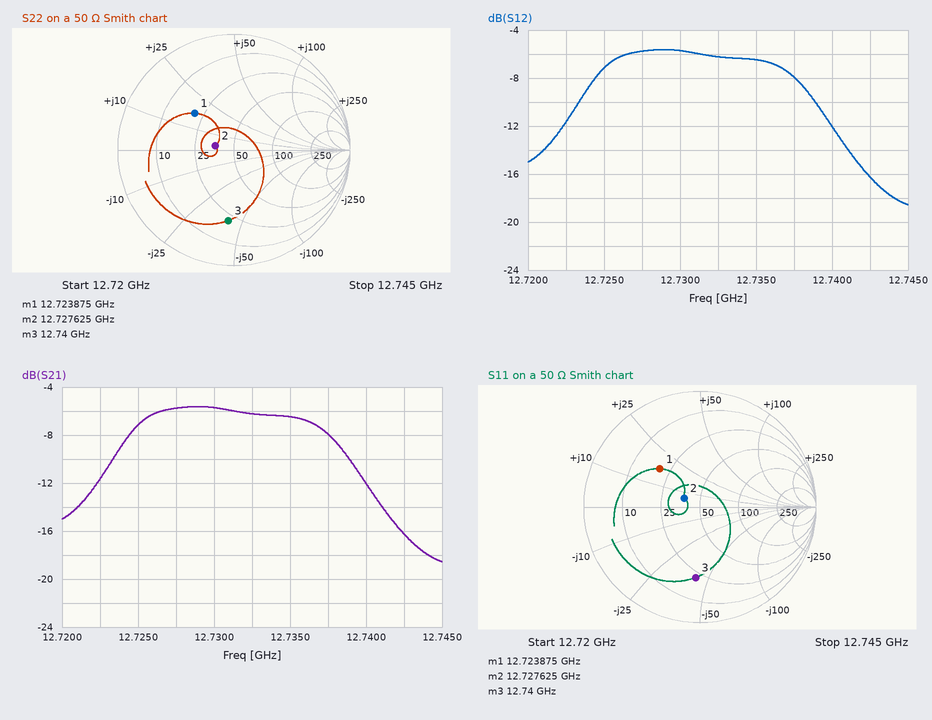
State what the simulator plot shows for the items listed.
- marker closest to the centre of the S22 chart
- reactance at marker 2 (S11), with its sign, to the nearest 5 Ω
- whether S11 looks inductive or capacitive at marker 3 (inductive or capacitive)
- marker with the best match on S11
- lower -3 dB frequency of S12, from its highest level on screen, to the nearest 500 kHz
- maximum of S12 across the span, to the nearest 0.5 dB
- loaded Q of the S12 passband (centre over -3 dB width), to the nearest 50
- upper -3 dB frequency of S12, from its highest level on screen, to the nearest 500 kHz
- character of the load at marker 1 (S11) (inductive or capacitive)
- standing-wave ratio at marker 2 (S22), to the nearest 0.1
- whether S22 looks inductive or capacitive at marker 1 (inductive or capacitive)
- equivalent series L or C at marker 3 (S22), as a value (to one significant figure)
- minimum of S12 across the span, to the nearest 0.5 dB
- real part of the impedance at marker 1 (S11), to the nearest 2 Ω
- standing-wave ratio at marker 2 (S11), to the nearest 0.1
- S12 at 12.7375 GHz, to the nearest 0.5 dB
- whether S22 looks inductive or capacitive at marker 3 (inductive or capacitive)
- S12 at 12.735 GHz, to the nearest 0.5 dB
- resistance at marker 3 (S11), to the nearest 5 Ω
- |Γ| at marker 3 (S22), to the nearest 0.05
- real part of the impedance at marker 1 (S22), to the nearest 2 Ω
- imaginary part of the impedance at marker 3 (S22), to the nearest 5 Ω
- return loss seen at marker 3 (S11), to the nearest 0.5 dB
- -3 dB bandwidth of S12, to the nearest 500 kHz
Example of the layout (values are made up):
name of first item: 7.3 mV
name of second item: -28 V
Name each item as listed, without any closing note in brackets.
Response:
marker closest to the centre of the S22 chart: marker 2
reactance at marker 2 (S11), with its sign, to the nearest 5 Ω: +5 Ω
whether S11 looks inductive or capacitive at marker 3: capacitive
marker with the best match on S11: marker 2
lower -3 dB frequency of S12, from its highest level on screen, to the nearest 500 kHz: 12.7240 GHz
maximum of S12 across the span, to the nearest 0.5 dB: -5.5 dB
loaded Q of the S12 passband (centre over -3 dB width), to the nearest 50: 900
upper -3 dB frequency of S12, from its highest level on screen, to the nearest 500 kHz: 12.7380 GHz
character of the load at marker 1 (S11): inductive
standing-wave ratio at marker 2 (S22), to the nearest 0.1: 1.4
whether S22 looks inductive or capacitive at marker 1: inductive
equivalent series L or C at marker 3 (S22), as a value: 300 fF
minimum of S12 across the span, to the nearest 0.5 dB: -18.5 dB
real part of the impedance at marker 1 (S11), to the nearest 2 Ω: 20 Ω
standing-wave ratio at marker 2 (S11), to the nearest 0.1: 1.4
S12 at 12.7375 GHz, to the nearest 0.5 dB: -8.0 dB
whether S22 looks inductive or capacitive at marker 3: capacitive
S12 at 12.735 GHz, to the nearest 0.5 dB: -6.5 dB
resistance at marker 3 (S11), to the nearest 5 Ω: 20 Ω
|Γ| at marker 3 (S22), to the nearest 0.05: 0.60
real part of the impedance at marker 1 (S22), to the nearest 2 Ω: 20 Ω
imaginary part of the impedance at marker 3 (S22), to the nearest 5 Ω: -40 Ω
return loss seen at marker 3 (S11), to the nearest 0.5 dB: 4.5 dB
-3 dB bandwidth of S12, to the nearest 500 kHz: 14.0 MHz
